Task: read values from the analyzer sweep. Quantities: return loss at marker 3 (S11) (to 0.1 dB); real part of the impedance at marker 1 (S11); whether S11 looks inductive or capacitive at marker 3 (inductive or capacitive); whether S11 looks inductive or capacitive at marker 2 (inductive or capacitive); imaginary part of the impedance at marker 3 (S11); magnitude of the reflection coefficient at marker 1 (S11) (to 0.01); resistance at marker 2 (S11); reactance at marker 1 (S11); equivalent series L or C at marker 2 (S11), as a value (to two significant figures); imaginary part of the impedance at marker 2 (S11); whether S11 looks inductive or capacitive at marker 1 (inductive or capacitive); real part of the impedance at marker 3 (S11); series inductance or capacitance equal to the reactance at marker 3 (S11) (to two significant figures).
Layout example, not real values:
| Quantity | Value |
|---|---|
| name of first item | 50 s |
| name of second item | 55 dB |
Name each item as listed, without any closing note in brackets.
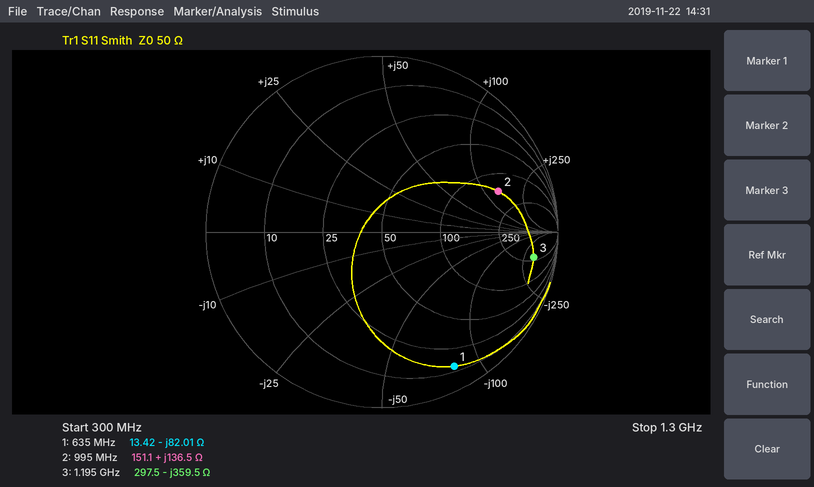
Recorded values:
| Quantity | Value |
|---|---|
| return loss at marker 3 (S11) | 1.2 dB |
| real part of the impedance at marker 1 | 13.42 Ω |
| whether S11 looks inductive or capacitive at marker 3 | capacitive |
| whether S11 looks inductive or capacitive at marker 2 | inductive |
| imaginary part of the impedance at marker 3 | -359.5 Ω |
| magnitude of the reflection coefficient at marker 1 (S11) | 0.87 |
| resistance at marker 2 | 151.1 Ω |
| reactance at marker 1 | -82.01 Ω |
| equivalent series L or C at marker 2 (S11), as a value | 22 nH |
| imaginary part of the impedance at marker 2 | +136.5 Ω |
| whether S11 looks inductive or capacitive at marker 1 | capacitive |
| real part of the impedance at marker 3 | 297.5 Ω |
| series inductance or capacitance equal to the reactance at marker 3 (S11) | 370 fF |
